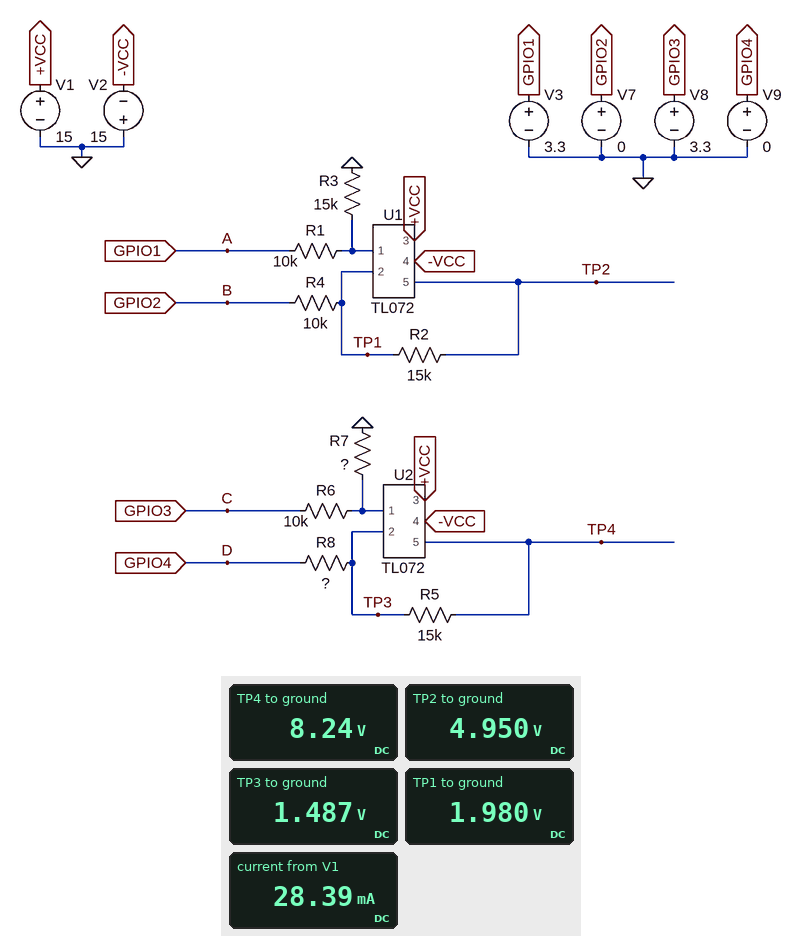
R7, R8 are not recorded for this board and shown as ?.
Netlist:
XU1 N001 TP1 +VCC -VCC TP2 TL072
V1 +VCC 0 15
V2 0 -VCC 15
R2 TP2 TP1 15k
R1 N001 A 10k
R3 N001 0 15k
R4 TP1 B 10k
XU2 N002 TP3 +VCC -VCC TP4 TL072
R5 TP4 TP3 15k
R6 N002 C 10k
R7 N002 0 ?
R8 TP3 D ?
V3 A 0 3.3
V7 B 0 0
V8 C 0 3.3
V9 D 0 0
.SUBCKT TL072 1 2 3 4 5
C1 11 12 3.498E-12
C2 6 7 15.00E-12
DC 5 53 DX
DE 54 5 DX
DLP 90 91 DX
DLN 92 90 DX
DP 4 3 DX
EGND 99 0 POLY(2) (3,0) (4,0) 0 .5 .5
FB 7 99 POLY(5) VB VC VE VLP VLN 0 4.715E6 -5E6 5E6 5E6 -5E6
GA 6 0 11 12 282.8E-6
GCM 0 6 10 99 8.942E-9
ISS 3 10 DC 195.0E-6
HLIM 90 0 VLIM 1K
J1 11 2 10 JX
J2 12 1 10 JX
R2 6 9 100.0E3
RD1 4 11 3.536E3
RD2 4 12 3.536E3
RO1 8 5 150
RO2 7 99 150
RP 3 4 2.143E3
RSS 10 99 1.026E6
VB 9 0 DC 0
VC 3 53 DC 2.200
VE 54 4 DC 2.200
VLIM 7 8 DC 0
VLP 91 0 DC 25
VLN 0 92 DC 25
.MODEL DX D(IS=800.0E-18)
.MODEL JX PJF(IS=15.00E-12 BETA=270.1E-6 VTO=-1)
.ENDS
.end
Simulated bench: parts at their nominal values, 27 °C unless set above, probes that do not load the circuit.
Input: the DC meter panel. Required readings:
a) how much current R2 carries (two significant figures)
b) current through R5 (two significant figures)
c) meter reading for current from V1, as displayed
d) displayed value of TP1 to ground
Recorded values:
200 µA
450 µA
28.39 mA
1.980 V
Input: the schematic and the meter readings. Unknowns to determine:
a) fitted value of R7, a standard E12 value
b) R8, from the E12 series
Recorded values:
8.2 kΩ
3.3 kΩ
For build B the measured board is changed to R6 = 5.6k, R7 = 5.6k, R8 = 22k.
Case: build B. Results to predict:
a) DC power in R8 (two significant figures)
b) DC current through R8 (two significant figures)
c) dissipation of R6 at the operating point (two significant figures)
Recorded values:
120 µW
75 µA
490 µW
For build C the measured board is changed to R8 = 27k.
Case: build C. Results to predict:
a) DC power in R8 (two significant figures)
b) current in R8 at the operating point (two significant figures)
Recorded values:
82 µW
55 µA
